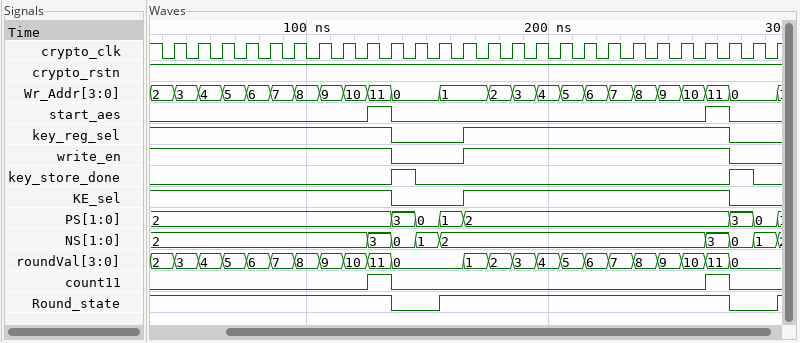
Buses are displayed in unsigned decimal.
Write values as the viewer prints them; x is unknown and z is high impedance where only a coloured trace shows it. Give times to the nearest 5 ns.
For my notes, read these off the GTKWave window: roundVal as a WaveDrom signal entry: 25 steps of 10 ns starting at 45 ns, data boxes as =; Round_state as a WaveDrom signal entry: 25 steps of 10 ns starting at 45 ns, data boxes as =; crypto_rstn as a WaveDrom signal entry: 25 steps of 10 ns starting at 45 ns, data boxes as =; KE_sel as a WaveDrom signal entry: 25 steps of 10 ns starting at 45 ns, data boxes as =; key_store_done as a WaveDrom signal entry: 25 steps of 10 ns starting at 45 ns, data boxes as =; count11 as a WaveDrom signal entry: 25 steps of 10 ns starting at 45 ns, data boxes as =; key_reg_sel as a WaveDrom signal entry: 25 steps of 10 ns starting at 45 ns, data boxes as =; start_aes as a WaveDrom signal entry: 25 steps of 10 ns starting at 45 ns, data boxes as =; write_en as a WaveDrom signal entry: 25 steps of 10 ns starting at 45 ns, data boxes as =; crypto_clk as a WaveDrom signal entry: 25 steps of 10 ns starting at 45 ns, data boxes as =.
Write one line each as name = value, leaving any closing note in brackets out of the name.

roundVal as a WaveDrom signal entry: 25 steps of 10 ns starting at 45 ns, data boxes as = = {name: 'roundVal', wave: '==========..============.', data: '3 4 5 6 7 8 9 10 11 0 1 2 3 4 5 6 7 8 9 10 11 0'}
Round_state as a WaveDrom signal entry: 25 steps of 10 ns starting at 45 ns, data boxes as = = {name: 'Round_state', wave: '1........0.1...........0.'}
crypto_rstn as a WaveDrom signal entry: 25 steps of 10 ns starting at 45 ns, data boxes as = = {name: 'crypto_rstn', wave: '1........................'}
KE_sel as a WaveDrom signal entry: 25 steps of 10 ns starting at 45 ns, data boxes as = = {name: 'KE_sel', wave: '1........0..1..........0.'}
key_store_done as a WaveDrom signal entry: 25 steps of 10 ns starting at 45 ns, data boxes as = = {name: 'key_store_done', wave: '0........10............10'}
count11 as a WaveDrom signal entry: 25 steps of 10 ns starting at 45 ns, data boxes as = = {name: 'count11', wave: '0.......10............10.'}
key_reg_sel as a WaveDrom signal entry: 25 steps of 10 ns starting at 45 ns, data boxes as = = {name: 'key_reg_sel', wave: '1........0..1..........0.'}
start_aes as a WaveDrom signal entry: 25 steps of 10 ns starting at 45 ns, data boxes as = = {name: 'start_aes', wave: '0.......10............10.'}
write_en as a WaveDrom signal entry: 25 steps of 10 ns starting at 45 ns, data boxes as = = {name: 'write_en', wave: '1........0..1..........0.'}
crypto_clk as a WaveDrom signal entry: 25 steps of 10 ns starting at 45 ns, data boxes as = = {name: 'crypto_clk', wave: 'p........................'}
